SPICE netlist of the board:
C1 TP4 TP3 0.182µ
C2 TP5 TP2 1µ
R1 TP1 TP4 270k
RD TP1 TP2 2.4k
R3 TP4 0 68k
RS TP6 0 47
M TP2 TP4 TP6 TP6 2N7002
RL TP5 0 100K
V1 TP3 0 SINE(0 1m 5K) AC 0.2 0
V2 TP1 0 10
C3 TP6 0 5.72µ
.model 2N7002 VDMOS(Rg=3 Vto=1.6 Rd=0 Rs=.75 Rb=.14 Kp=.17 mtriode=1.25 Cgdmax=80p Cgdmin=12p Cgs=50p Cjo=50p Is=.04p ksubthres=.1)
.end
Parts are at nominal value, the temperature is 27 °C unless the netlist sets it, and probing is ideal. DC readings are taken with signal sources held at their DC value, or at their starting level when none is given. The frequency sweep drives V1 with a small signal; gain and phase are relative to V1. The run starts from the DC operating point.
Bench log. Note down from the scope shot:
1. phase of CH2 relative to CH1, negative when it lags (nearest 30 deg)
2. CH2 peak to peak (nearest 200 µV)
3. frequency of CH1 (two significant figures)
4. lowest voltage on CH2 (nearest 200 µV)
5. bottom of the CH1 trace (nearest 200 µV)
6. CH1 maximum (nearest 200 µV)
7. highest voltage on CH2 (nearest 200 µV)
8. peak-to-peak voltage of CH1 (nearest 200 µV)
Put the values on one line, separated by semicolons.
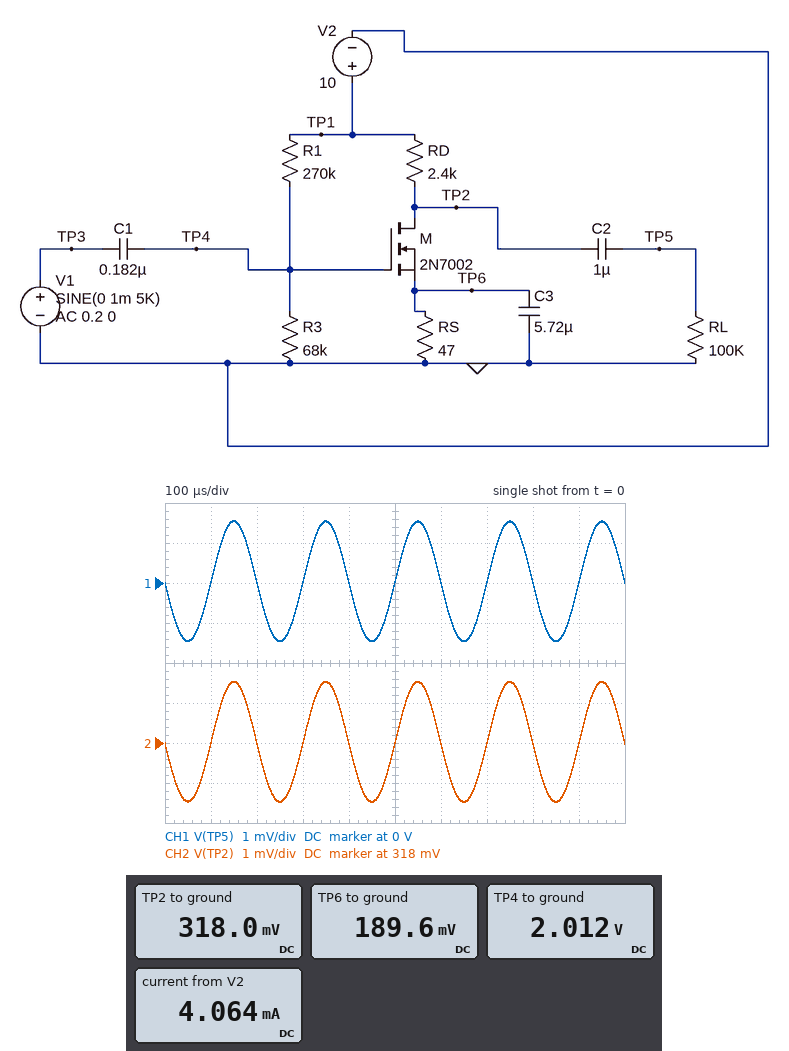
0 deg; 3.0 mV; 5.0 kHz; 316.6 mV; -1.4 mV; 1.6 mV; 319.6 mV; 3.0 mV
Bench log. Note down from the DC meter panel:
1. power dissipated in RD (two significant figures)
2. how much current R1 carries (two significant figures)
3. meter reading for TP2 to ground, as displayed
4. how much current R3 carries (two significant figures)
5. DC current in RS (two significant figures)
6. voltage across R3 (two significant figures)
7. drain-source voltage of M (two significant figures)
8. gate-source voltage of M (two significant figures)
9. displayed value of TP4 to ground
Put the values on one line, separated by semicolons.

39 mW; 30 µA; 318.0 mV; 30 µA; 4.0 mA; 2.0 V; 130 mV; 1.8 V; 2.012 V
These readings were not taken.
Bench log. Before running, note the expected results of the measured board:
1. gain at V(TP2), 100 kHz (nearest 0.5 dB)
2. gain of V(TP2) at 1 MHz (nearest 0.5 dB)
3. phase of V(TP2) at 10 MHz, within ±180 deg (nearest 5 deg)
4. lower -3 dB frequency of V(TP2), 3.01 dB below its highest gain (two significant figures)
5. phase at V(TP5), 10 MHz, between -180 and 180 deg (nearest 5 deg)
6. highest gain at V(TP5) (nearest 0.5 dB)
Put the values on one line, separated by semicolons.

3.5 dB; 3.5 dB; 140 deg; 18 Hz; 140 deg; 3.5 dB
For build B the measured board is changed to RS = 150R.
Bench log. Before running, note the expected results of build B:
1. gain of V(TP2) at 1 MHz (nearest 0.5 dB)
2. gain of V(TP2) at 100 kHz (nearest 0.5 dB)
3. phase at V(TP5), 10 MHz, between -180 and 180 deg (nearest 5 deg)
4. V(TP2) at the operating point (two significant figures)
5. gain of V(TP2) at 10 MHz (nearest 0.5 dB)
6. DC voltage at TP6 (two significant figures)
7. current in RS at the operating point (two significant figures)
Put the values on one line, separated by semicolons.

32.0 dB; 33.0 dB; 95 deg; 5.4 V; 18.0 dB; 290 mV; 1.9 mA
